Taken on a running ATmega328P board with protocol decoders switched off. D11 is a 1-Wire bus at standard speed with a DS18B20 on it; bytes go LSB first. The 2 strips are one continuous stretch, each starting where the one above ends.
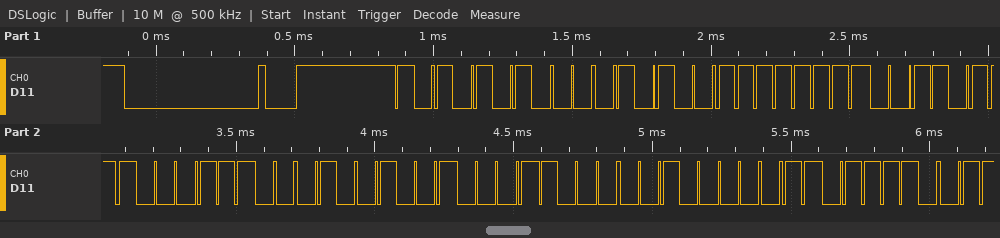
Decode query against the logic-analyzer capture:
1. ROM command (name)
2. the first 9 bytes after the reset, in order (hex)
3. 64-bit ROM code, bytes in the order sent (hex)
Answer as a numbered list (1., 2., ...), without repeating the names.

1. Match ROM
2. 55 28 FF EC 38 92 18 04 7B
3. 28 FF EC 38 92 18 04 7B
